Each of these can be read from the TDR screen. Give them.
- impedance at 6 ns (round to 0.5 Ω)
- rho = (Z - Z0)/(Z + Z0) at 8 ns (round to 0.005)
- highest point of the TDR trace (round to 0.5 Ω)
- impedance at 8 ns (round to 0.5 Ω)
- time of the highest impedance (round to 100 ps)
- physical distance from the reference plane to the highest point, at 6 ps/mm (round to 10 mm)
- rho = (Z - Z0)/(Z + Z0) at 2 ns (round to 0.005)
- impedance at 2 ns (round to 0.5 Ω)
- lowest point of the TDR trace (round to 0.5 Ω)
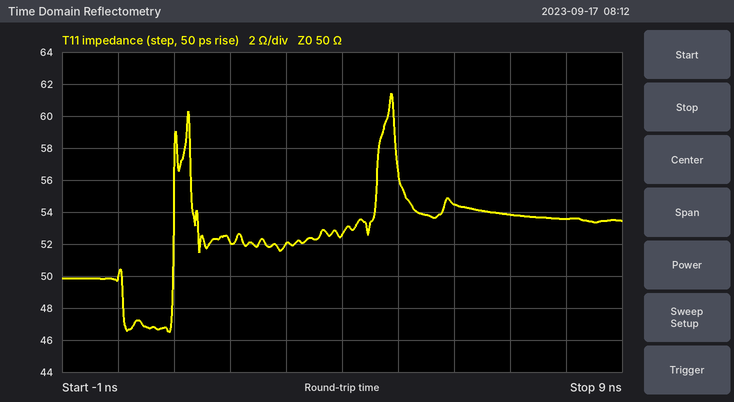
54.5 Ω
+0.035
61.5 Ω
53.5 Ω
4.9 ns
410 mm
+0.020
52.0 Ω
46.5 Ω
